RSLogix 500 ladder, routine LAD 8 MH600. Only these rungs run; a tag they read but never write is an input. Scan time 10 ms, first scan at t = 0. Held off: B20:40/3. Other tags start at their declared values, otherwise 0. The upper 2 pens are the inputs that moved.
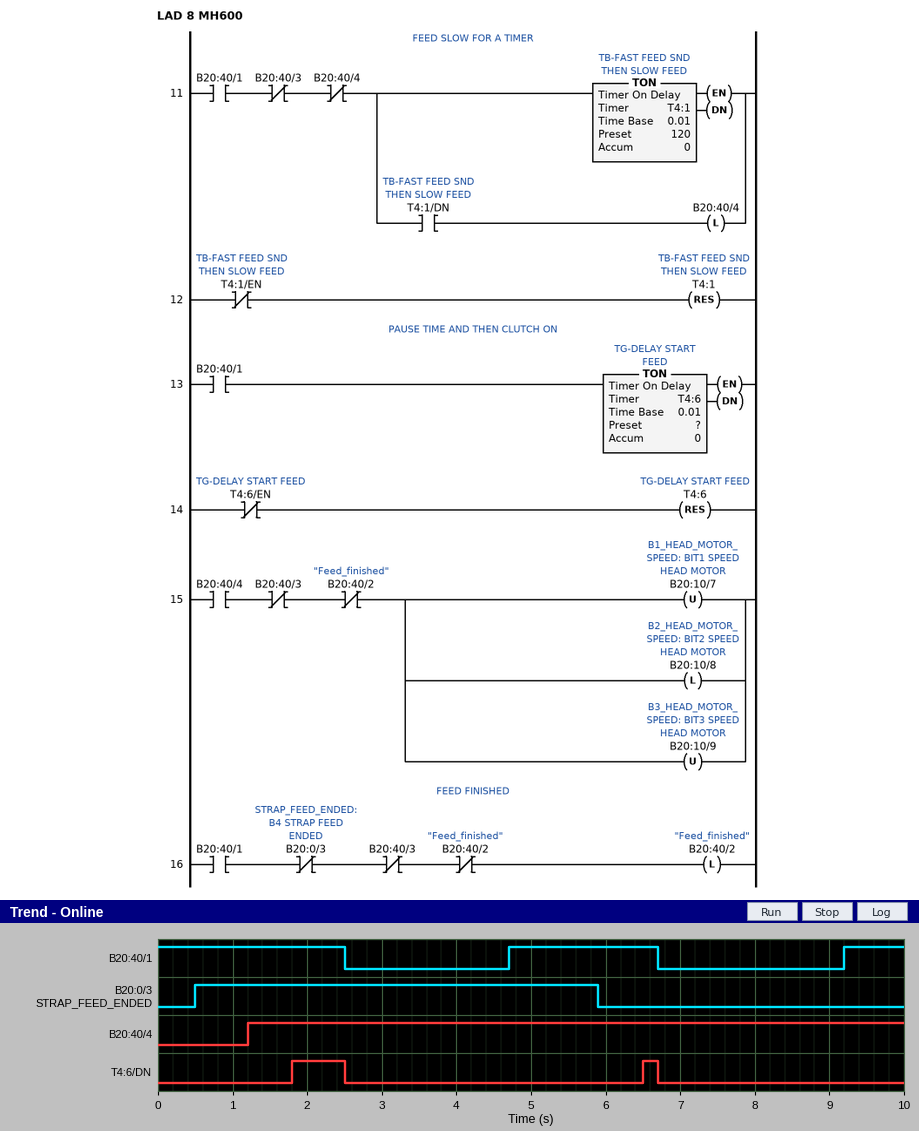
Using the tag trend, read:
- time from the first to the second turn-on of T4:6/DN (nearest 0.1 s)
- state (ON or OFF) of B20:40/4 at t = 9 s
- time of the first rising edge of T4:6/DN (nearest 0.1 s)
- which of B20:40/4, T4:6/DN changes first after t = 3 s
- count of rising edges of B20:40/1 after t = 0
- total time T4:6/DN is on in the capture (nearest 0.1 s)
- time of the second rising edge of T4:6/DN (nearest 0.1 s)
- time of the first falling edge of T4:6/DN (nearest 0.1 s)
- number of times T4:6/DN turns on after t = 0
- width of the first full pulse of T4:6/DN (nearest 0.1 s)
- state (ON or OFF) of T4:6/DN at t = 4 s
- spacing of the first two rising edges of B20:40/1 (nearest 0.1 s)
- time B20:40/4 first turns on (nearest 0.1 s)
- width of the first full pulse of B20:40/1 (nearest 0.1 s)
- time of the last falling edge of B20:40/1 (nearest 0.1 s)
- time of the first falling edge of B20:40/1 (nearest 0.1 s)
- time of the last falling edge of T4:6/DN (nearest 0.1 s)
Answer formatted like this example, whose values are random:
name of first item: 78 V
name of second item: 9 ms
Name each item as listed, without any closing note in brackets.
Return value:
time from the first to the second turn-on of T4:6/DN: 4.7 s
state (ON or OFF) of B20:40/4 at t = 9 s: ON
time of the first rising edge of T4:6/DN: 1.8 s
which of B20:40/4, T4:6/DN changes first after t = 3 s: T4:6/DN
count of rising edges of B20:40/1 after t = 0: 2
total time T4:6/DN is on in the capture: 0.9 s
time of the second rising edge of T4:6/DN: 6.5 s
time of the first falling edge of T4:6/DN: 2.5 s
number of times T4:6/DN turns on after t = 0: 2
width of the first full pulse of T4:6/DN: 0.7 s
state (ON or OFF) of T4:6/DN at t = 4 s: OFF
spacing of the first two rising edges of B20:40/1: 4.5 s
time B20:40/4 first turns on: 1.2 s
width of the first full pulse of B20:40/1: 2.0 s
time of the last falling edge of B20:40/1: 6.7 s
time of the first falling edge of B20:40/1: 2.5 s
time of the last falling edge of T4:6/DN: 6.7 s
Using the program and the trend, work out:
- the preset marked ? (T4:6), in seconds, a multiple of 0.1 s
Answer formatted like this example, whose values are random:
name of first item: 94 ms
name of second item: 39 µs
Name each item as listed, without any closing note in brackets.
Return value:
the preset marked ? (T4:6), in seconds, a multiple of 0.1 s: 1.8 s
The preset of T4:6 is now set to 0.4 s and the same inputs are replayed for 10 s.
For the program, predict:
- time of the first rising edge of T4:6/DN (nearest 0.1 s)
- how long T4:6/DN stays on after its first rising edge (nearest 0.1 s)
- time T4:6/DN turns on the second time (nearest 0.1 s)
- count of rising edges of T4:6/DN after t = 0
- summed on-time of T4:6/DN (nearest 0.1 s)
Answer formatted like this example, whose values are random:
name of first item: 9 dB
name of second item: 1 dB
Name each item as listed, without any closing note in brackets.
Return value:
time of the first rising edge of T4:6/DN: 0.4 s
how long T4:6/DN stays on after its first rising edge: 2.1 s
time T4:6/DN turns on the second time: 5.1 s
count of rising edges of T4:6/DN after t = 0: 3
summed on-time of T4:6/DN: 4.1 s
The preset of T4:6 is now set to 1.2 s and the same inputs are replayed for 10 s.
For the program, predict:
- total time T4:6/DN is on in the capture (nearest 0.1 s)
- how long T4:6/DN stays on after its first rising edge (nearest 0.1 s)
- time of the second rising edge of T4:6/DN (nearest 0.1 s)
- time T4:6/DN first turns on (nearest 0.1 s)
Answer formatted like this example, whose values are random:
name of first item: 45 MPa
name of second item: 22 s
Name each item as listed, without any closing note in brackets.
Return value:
total time T4:6/DN is on in the capture: 2.1 s
how long T4:6/DN stays on after its first rising edge: 1.3 s
time of the second rising edge of T4:6/DN: 5.9 s
time T4:6/DN first turns on: 1.2 s
